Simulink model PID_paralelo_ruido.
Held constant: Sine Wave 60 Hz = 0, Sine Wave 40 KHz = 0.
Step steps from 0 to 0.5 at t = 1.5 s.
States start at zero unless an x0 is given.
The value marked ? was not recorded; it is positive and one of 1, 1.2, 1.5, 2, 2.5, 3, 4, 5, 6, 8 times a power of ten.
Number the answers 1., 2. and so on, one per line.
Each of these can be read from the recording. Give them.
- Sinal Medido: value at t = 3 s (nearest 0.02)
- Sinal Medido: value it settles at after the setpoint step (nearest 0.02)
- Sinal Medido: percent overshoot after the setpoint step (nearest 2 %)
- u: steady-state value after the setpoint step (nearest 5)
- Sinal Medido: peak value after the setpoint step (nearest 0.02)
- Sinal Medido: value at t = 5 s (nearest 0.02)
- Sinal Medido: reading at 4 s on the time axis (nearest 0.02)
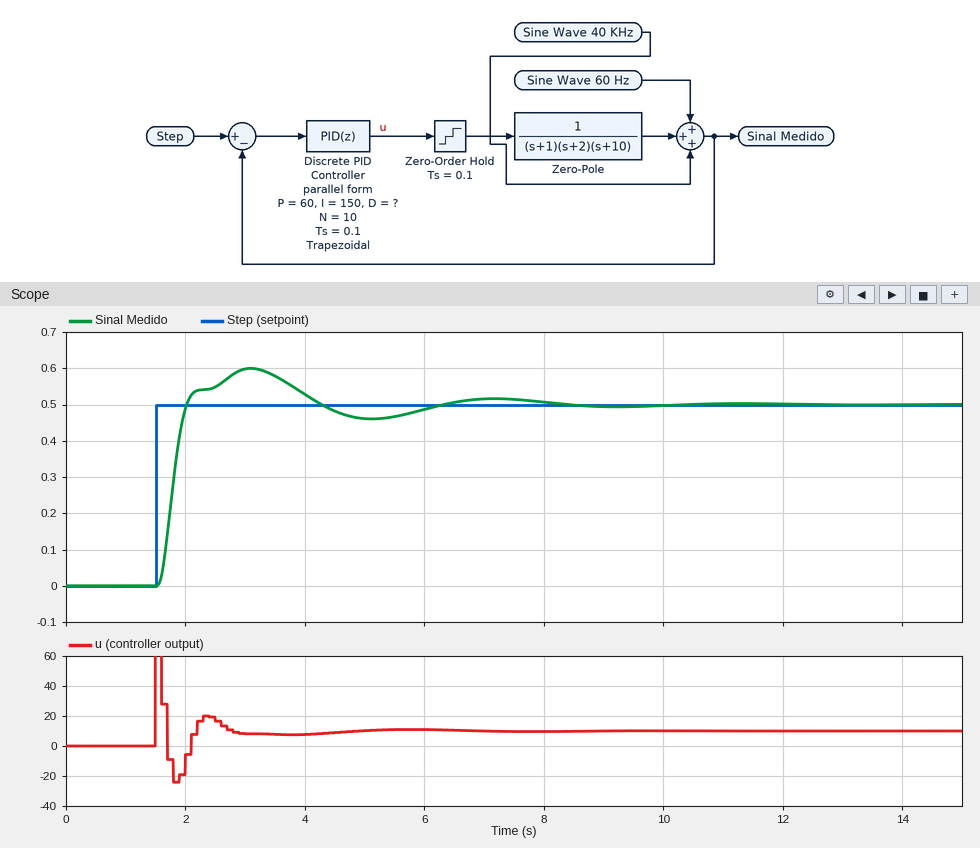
1. 0.60
2. 0.50
3. 20 %
4. 10
5. 0.60
6. 0.46
7. 0.52
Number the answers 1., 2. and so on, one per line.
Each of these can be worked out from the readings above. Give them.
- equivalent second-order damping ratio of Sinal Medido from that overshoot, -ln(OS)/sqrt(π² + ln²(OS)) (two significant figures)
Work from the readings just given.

1. 0.46
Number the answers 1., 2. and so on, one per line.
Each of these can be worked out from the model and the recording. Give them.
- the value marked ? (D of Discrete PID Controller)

1. 40
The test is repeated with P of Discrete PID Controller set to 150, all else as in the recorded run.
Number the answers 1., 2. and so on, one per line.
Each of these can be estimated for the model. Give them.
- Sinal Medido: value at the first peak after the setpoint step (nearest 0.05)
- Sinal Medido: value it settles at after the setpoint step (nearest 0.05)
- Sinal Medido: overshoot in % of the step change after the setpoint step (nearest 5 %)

1. 0.70
2. 0.50
3. 40 %
